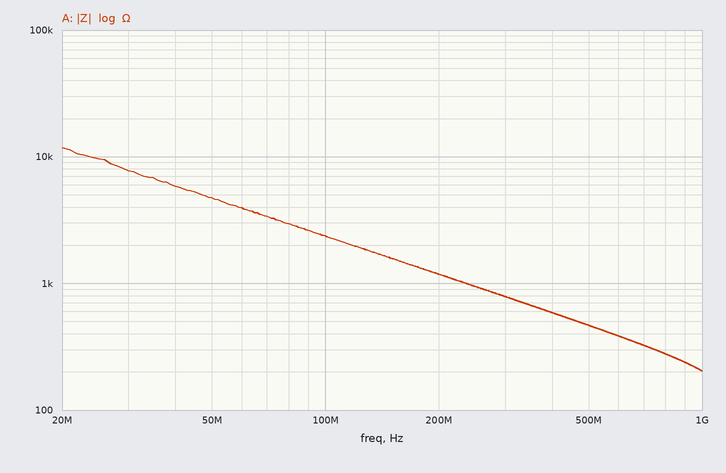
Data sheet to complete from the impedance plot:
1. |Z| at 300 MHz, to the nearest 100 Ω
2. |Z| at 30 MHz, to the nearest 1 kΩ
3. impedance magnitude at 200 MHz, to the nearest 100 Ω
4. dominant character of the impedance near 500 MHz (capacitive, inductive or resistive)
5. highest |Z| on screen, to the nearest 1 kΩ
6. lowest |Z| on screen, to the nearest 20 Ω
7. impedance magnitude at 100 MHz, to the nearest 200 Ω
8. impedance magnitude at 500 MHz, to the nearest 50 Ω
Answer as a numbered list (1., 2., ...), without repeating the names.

1. 800 Ω
2. 8 kΩ
3. 1.2 kΩ
4. capacitive
5. 12 kΩ
6. 200 Ω
7. 2.4 kΩ
8. 450 Ω
